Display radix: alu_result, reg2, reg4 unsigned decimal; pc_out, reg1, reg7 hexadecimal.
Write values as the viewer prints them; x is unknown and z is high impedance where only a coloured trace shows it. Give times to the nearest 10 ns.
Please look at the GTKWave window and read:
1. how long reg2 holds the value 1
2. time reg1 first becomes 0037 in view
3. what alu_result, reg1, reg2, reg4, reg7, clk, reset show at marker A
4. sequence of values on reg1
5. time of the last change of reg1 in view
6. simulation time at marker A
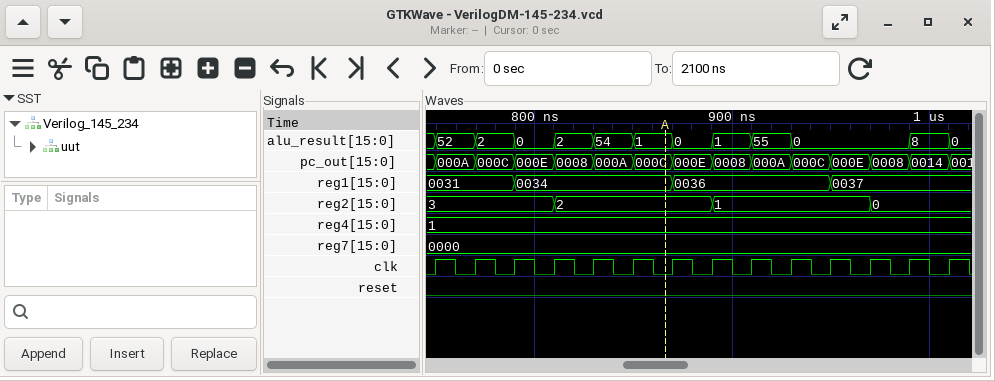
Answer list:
80 ns
950 ns
alu_result=1, reg1=0034, reg2=2, reg4=1, reg7=0000, clk=0, reset=0
0031, 0034, 0036, 0037
950 ns
870 ns
